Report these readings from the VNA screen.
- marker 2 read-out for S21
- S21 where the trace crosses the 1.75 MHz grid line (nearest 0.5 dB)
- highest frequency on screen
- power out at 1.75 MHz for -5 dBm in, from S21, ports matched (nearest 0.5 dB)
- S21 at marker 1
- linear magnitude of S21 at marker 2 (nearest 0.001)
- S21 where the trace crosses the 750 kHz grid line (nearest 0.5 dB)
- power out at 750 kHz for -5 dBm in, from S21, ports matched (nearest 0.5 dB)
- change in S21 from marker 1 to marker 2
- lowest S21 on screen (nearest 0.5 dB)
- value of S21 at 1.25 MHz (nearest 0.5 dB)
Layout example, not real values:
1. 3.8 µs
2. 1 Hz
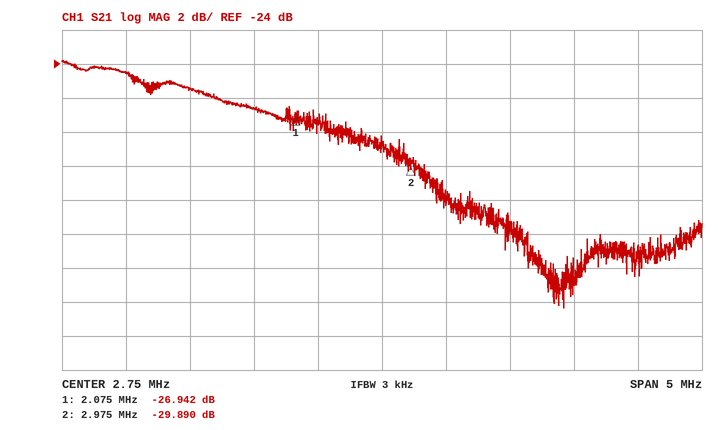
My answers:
1. -29.890 dB
2. -26.5 dB
3. 5.25 MHz
4. -31.5 dBm
5. -26.942 dB
6. 0.032
7. -24.5 dB
8. -29.5 dBm
9. -2.948 dB
10. -38.5 dB
11. -25.5 dB
